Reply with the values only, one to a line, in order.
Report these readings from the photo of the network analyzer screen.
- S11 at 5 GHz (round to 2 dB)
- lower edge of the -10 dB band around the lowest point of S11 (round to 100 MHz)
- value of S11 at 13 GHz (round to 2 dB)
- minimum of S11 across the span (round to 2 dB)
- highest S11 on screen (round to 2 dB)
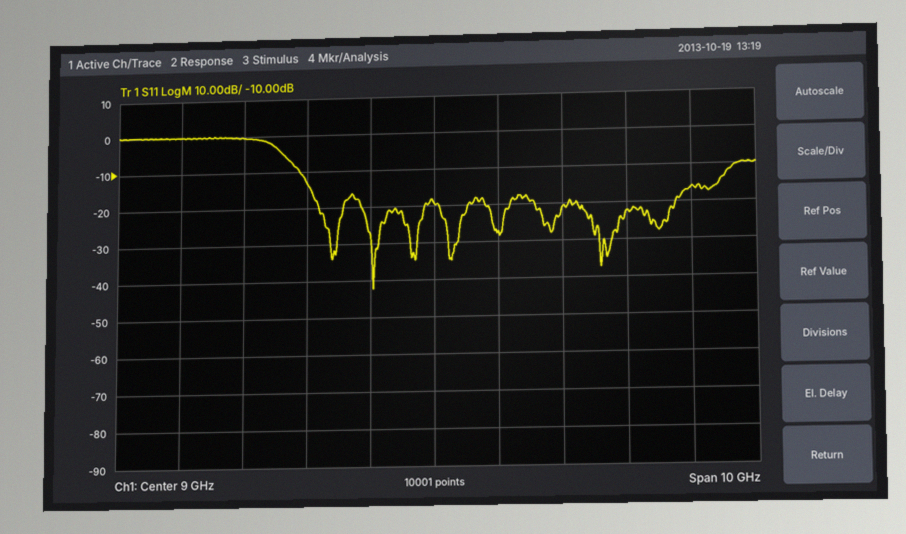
0 dB
6.9 GHz
-16 dB
-42 dB
0 dB
